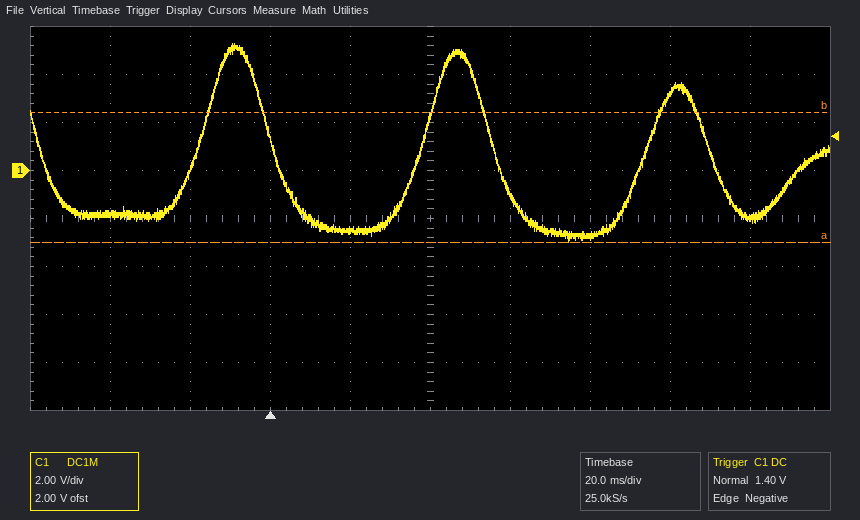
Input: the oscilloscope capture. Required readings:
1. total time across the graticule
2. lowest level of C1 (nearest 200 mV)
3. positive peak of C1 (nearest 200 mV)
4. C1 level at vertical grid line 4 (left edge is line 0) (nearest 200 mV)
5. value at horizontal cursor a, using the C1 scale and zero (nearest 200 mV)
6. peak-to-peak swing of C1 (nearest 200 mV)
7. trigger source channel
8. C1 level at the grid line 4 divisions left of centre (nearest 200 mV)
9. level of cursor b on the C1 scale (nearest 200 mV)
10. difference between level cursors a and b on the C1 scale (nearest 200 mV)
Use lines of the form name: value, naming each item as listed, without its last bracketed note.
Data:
total time across the graticule: 200 ms
lowest level of C1: -3.0 V
positive peak of C1: 5.2 V
C1 level at vertical grid line 4 (left edge is line 0): -2.4 V
value at horizontal cursor a, using the C1 scale and zero: -3.0 V
peak-to-peak swing of C1: 8.2 V
trigger source channel: C1
C1 level at the grid line 4 divisions left of centre: -1.8 V
level of cursor b on the C1 scale: 2.4 V
difference between level cursors a and b on the C1 scale: 5.4 V
